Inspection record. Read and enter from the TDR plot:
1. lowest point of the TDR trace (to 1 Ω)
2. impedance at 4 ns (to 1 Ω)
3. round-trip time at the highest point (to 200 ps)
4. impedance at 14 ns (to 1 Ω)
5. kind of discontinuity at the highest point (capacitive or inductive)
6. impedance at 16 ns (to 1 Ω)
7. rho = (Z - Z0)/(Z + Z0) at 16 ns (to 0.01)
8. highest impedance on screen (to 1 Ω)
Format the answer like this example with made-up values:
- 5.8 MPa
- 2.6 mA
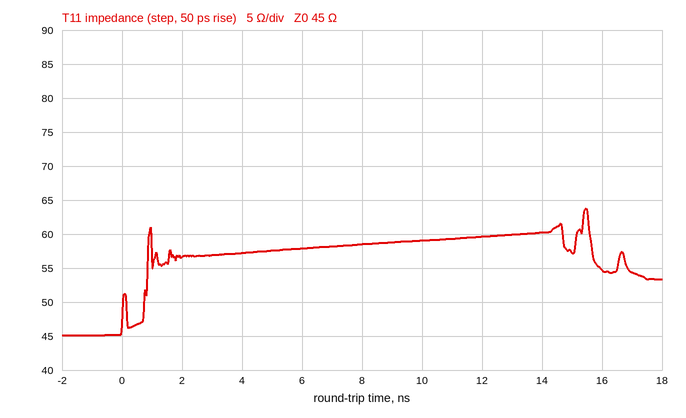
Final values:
- 45 Ω
- 57 Ω
- 15.4 ns
- 60 Ω
- inductive
- 55 Ω
- +0.10
- 64 Ω
